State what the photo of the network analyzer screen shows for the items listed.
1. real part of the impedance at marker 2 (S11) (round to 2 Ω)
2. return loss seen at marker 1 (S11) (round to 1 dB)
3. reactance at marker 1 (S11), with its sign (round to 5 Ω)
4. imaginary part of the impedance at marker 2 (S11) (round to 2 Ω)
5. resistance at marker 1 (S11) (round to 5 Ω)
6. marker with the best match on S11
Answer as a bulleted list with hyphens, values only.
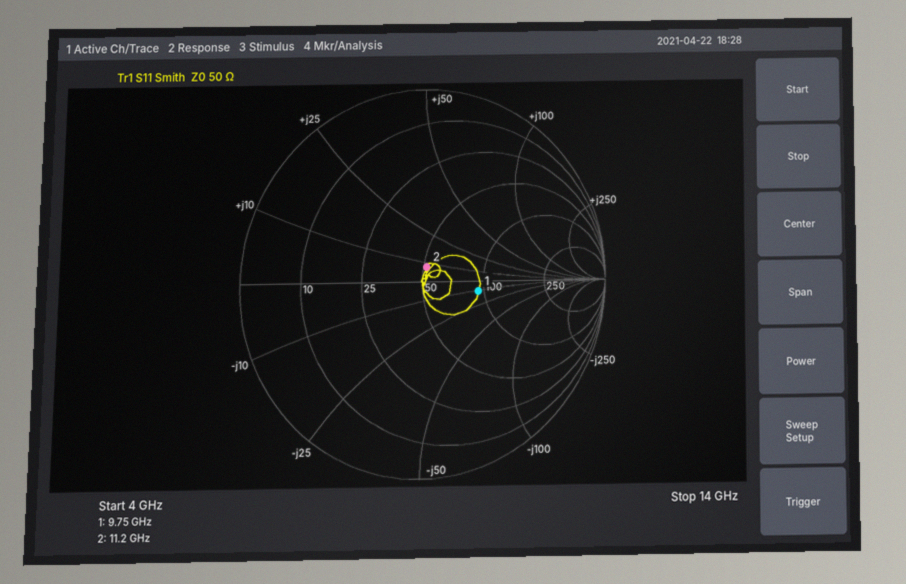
- 52 Ω
- 10 dB
- -10 Ω
- +8 Ω
- 95 Ω
- marker 2
